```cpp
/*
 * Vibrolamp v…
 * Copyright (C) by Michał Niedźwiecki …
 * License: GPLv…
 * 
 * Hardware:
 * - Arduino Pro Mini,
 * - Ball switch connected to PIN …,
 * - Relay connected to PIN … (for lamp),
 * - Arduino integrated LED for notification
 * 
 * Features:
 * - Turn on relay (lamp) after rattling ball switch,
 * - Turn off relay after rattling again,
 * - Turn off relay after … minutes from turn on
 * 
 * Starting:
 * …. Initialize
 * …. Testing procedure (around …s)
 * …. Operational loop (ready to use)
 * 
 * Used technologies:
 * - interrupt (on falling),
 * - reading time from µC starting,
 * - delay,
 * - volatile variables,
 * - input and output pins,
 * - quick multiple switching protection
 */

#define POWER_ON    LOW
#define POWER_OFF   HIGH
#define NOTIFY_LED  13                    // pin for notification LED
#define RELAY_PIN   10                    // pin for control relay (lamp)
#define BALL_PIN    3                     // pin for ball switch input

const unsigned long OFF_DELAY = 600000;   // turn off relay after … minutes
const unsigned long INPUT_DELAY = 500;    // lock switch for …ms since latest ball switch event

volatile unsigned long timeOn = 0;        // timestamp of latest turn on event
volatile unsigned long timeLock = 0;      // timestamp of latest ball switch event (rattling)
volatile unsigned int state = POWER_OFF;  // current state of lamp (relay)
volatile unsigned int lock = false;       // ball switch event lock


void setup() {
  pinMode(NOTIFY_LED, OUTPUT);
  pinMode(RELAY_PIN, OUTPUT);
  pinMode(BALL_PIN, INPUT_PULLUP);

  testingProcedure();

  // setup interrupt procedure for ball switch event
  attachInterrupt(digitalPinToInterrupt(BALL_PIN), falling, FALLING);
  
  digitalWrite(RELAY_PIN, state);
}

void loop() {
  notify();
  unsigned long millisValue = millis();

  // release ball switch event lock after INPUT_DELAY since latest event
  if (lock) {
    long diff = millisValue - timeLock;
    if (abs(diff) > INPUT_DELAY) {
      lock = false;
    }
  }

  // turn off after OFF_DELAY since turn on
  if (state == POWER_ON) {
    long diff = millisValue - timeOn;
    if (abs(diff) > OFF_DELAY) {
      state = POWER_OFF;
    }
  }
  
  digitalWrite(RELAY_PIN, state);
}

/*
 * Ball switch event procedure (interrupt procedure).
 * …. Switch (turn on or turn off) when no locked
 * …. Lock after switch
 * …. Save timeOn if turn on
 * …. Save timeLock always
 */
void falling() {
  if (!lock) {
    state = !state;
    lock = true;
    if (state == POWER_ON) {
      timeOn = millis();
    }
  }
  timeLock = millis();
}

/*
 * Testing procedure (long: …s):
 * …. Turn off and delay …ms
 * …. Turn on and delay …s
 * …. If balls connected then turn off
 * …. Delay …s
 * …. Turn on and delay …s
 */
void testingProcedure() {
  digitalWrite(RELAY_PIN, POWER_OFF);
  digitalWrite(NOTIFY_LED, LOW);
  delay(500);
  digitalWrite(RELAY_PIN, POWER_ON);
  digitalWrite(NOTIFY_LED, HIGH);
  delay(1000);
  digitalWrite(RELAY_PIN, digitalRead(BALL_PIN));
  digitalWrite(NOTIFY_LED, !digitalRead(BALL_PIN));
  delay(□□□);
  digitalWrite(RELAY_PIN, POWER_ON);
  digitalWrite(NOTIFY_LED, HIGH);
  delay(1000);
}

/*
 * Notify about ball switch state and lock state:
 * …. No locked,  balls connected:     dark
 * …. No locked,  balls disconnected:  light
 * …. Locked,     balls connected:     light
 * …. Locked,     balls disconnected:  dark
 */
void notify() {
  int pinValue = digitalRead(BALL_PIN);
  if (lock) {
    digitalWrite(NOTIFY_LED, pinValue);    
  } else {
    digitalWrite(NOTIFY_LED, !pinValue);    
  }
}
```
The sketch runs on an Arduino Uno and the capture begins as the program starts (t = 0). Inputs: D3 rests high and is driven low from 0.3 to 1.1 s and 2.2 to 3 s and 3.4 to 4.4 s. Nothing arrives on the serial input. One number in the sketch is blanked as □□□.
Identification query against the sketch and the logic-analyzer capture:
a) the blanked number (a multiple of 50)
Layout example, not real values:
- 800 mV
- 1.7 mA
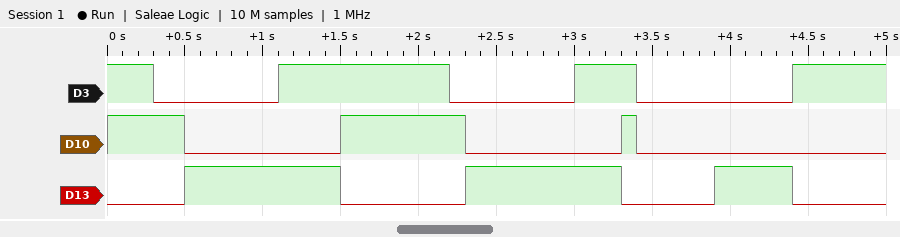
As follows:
- 800
